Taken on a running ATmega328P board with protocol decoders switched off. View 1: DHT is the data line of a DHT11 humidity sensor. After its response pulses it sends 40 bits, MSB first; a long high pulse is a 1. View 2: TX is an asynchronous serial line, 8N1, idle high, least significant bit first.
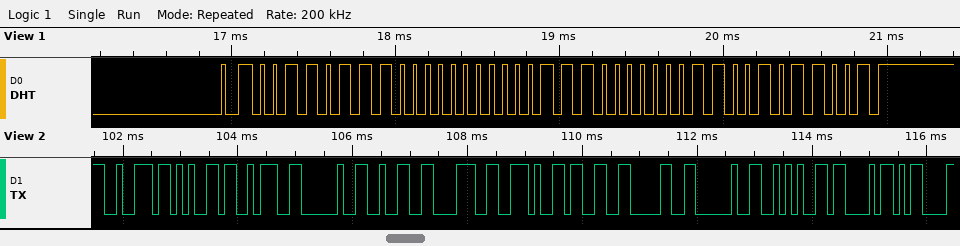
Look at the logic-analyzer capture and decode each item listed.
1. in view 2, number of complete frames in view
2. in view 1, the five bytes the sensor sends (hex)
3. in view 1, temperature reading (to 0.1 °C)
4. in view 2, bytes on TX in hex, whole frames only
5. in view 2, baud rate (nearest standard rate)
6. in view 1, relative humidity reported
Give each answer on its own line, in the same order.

13
37 00 1C 06 59
28.6 °C
0x72 0x65 0x3A 0x20 0x32 0x38 0x2E 0x33 0x30 0x20 0x2A 0x43 0x0D
9600 baud
55 %
